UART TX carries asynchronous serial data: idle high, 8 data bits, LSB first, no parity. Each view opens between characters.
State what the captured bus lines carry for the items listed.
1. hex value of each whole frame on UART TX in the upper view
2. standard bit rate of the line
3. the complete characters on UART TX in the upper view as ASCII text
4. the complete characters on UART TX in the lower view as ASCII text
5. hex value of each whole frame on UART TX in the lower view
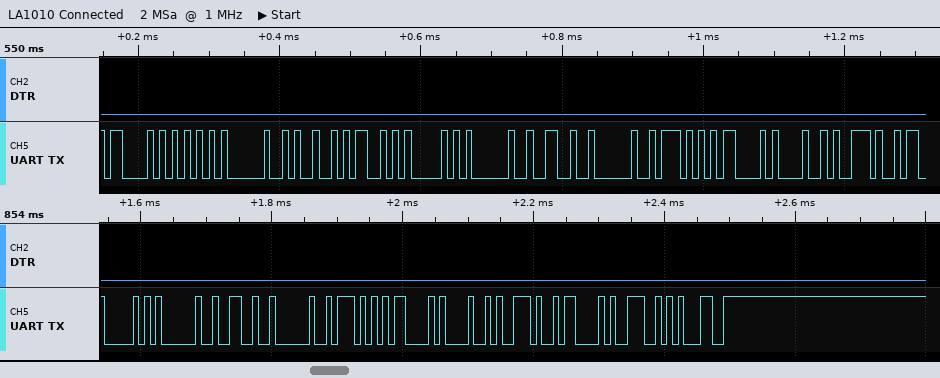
43, 55, 20, 49, 53, 50, 20, 26, 20, 57, 43, 48, 2E
115200 baud
"CU ISP & WCH."
"P & WCH.CN1"
50, 20, 26, 20, 57, 43, 48, 2E, 43, 4E, 31
